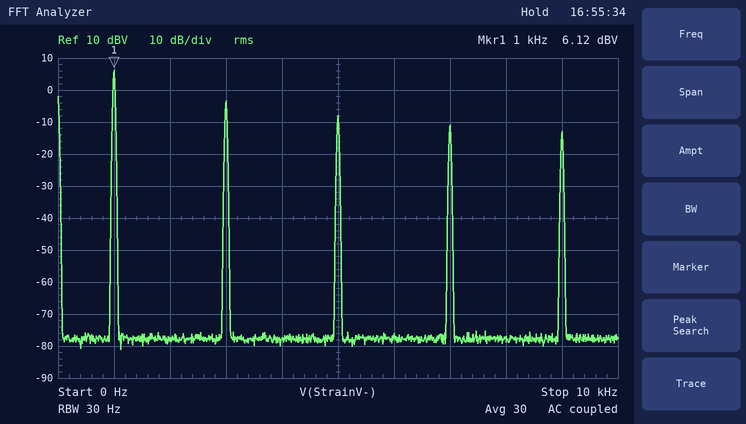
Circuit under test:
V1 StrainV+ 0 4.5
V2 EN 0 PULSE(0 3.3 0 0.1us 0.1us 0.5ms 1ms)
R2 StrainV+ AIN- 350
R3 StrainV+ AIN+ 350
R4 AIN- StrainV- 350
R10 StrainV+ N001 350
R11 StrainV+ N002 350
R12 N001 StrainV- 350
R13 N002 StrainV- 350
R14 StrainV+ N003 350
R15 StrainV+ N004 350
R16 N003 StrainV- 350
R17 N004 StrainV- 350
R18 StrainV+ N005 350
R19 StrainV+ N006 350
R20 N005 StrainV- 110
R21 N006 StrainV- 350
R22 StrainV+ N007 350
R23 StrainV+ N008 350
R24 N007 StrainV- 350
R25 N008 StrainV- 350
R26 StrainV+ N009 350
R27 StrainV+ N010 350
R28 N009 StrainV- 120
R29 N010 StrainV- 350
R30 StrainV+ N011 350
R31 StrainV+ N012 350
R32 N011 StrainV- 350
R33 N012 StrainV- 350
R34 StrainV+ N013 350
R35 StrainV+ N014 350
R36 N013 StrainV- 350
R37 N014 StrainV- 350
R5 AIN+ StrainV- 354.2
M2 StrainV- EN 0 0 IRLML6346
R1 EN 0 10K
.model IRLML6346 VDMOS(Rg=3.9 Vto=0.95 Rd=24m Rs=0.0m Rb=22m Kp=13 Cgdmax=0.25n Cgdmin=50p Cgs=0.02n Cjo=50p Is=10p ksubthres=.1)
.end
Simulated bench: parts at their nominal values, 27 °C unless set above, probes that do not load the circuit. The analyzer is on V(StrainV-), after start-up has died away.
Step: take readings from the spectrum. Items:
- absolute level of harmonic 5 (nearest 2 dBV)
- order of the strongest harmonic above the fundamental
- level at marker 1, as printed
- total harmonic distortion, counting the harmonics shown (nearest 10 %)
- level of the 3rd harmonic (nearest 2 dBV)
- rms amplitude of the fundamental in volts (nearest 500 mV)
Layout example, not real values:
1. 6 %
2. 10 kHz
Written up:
1. -8 dBV
2. 3
3. 6.12 dBV
4. 40 %
5. -4 dBV
6. 2.0 V
